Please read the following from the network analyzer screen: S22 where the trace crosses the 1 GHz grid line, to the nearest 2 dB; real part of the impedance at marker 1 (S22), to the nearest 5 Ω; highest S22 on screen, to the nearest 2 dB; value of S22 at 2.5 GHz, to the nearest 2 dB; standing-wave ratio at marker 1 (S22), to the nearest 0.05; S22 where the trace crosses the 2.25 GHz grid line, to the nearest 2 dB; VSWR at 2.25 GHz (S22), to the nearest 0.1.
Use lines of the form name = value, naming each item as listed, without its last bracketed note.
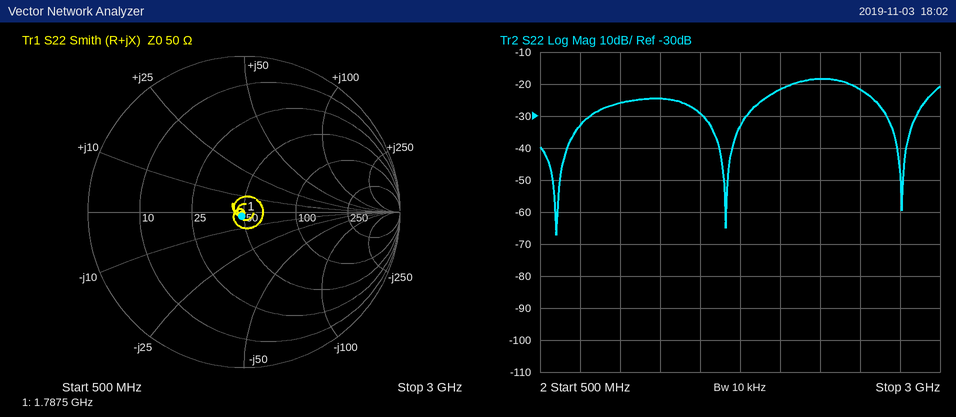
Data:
S22 where the trace crosses the 1 GHz grid line, to the nearest 2 dB = -26 dB
real part of the impedance at marker 1 (S22), to the nearest 5 Ω = 50 Ω
highest S22 on screen, to the nearest 2 dB = -18 dB
value of S22 at 2.5 GHz, to the nearest 2 dB = -22 dB
standing-wave ratio at marker 1 (S22), to the nearest 0.05 = 1.05
S22 where the trace crosses the 2.25 GHz grid line, to the nearest 2 dB = -18 dB
VSWR at 2.25 GHz (S22), to the nearest 0.1 = 1.3
